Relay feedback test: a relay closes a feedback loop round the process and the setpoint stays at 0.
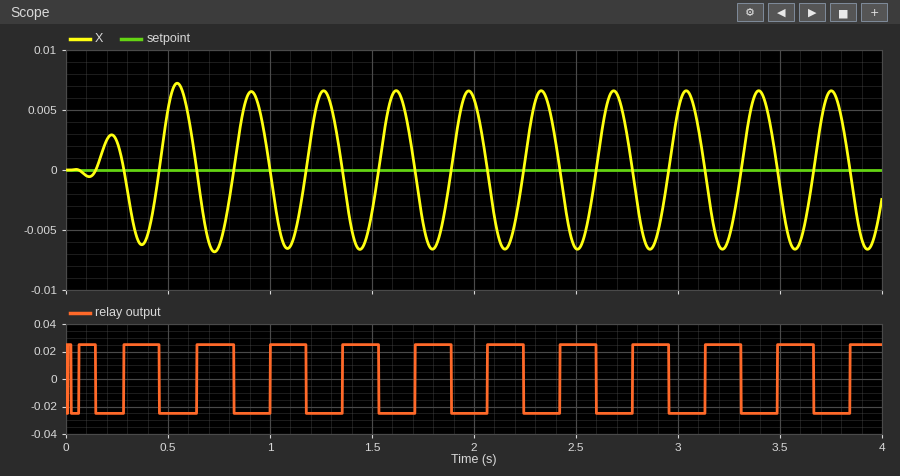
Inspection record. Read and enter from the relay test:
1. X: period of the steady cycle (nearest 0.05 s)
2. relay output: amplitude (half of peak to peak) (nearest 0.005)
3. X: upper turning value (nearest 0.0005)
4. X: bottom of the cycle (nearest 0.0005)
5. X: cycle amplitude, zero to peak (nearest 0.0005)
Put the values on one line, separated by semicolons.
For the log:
0.35 s; 0.025; 0.0065; -0.0065; 0.0065
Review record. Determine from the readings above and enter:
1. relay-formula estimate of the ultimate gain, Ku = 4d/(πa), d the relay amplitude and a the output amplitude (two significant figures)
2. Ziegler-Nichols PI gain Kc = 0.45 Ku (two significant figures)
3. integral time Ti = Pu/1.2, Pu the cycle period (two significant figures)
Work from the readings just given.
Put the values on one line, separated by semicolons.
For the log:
4.9; 2.2; 0.29 s
